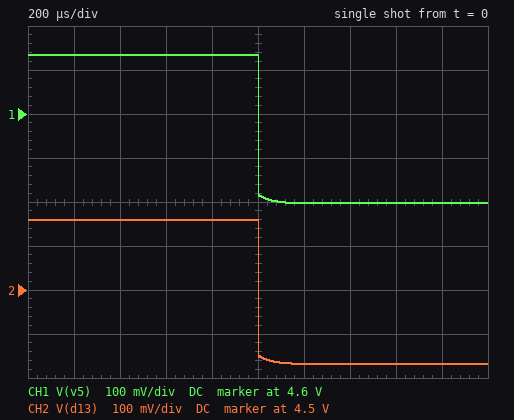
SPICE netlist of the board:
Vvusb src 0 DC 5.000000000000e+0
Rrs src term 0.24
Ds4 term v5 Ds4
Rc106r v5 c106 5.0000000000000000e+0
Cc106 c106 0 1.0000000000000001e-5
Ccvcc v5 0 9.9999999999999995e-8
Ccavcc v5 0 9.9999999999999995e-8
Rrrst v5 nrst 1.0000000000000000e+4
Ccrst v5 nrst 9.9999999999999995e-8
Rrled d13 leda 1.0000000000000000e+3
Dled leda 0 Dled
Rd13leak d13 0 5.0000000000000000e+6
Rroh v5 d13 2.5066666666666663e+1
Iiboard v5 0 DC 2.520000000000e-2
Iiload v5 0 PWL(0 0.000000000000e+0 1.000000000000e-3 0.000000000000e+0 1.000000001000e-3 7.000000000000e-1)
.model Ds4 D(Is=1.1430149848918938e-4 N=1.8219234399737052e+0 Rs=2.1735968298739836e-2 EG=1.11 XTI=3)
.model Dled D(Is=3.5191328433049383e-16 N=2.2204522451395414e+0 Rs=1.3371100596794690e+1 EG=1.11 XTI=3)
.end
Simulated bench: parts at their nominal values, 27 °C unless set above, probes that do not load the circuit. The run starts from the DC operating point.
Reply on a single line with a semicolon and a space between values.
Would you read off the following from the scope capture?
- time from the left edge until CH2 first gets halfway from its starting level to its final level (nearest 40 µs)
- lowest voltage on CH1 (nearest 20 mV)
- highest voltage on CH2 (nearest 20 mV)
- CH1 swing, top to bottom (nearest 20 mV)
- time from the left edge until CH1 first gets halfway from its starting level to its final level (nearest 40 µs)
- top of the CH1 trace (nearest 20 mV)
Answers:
1.00 ms; 4.40 V; 4.66 V; 340 mV; 1.00 ms; 4.74 V
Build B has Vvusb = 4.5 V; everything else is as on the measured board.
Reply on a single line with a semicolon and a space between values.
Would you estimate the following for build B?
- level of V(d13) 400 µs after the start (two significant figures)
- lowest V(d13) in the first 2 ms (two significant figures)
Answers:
4.2 V; 3.8 V
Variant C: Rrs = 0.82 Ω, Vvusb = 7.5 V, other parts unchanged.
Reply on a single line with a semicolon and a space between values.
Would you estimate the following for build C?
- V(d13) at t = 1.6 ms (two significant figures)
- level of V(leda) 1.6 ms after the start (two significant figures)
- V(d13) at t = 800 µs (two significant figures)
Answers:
6.4 V; 1.8 V; 7.1 V
